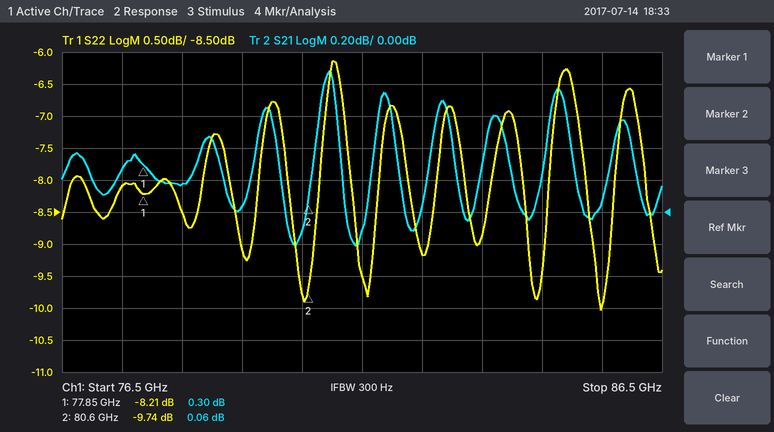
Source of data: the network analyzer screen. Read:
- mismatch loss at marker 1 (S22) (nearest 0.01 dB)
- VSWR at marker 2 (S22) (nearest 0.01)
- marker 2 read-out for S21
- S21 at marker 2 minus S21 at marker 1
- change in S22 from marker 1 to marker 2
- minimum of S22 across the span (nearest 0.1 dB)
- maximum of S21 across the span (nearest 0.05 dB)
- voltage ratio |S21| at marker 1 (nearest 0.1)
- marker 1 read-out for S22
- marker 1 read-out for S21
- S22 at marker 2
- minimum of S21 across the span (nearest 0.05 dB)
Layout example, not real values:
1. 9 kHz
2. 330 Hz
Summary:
1. 0.71 dB
2. 1.97
3. 0.06 dB
4. -0.24 dB
5. -1.53 dB
6. -10.0 dB
7. 0.90 dB
8. 1.0
9. -8.21 dB
10. 0.30 dB
11. -9.74 dB
12. -0.20 dB
